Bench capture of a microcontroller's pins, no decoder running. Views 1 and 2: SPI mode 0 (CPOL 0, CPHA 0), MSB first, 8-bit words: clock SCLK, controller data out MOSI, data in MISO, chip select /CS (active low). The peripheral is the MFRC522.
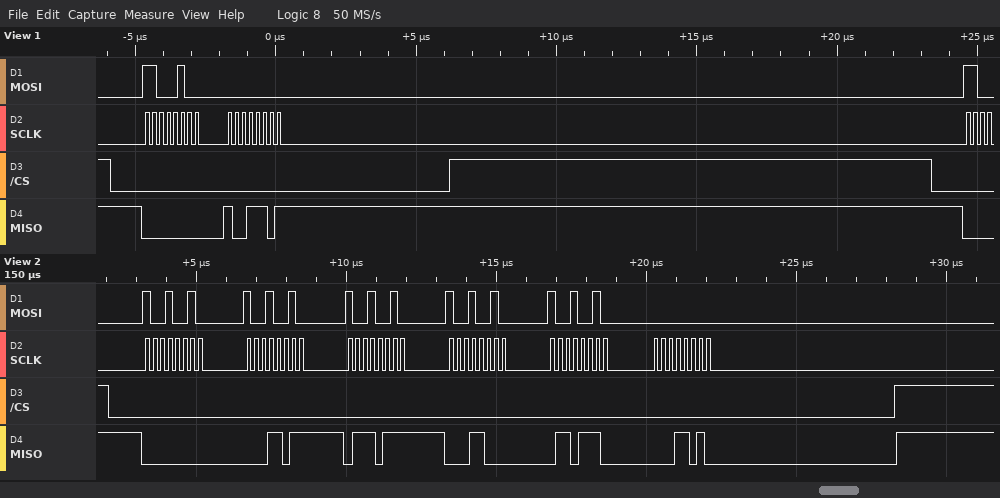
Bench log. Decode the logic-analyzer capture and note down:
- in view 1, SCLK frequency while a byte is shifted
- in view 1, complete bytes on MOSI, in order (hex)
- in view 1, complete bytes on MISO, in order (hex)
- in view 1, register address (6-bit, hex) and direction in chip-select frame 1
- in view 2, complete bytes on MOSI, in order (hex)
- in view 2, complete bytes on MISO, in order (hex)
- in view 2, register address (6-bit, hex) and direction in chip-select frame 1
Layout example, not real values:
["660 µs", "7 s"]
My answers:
["4 MHz", "0xC4 0x00", "0x00 0x9D", "0x22 read", "0x92 0x92 0x92 0x92 0x92 0x00", "0x00 0x1B 0x77 0x18 0x6E 0x1A", "0x09 read"]
